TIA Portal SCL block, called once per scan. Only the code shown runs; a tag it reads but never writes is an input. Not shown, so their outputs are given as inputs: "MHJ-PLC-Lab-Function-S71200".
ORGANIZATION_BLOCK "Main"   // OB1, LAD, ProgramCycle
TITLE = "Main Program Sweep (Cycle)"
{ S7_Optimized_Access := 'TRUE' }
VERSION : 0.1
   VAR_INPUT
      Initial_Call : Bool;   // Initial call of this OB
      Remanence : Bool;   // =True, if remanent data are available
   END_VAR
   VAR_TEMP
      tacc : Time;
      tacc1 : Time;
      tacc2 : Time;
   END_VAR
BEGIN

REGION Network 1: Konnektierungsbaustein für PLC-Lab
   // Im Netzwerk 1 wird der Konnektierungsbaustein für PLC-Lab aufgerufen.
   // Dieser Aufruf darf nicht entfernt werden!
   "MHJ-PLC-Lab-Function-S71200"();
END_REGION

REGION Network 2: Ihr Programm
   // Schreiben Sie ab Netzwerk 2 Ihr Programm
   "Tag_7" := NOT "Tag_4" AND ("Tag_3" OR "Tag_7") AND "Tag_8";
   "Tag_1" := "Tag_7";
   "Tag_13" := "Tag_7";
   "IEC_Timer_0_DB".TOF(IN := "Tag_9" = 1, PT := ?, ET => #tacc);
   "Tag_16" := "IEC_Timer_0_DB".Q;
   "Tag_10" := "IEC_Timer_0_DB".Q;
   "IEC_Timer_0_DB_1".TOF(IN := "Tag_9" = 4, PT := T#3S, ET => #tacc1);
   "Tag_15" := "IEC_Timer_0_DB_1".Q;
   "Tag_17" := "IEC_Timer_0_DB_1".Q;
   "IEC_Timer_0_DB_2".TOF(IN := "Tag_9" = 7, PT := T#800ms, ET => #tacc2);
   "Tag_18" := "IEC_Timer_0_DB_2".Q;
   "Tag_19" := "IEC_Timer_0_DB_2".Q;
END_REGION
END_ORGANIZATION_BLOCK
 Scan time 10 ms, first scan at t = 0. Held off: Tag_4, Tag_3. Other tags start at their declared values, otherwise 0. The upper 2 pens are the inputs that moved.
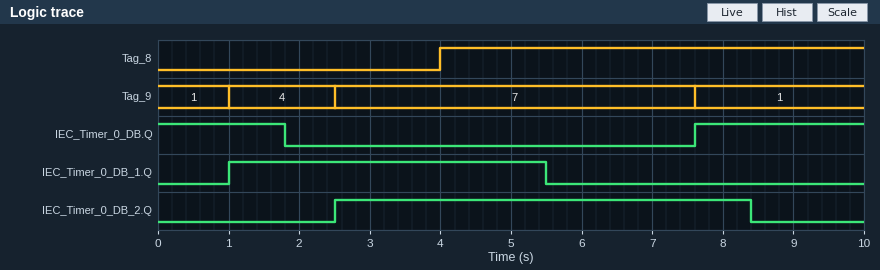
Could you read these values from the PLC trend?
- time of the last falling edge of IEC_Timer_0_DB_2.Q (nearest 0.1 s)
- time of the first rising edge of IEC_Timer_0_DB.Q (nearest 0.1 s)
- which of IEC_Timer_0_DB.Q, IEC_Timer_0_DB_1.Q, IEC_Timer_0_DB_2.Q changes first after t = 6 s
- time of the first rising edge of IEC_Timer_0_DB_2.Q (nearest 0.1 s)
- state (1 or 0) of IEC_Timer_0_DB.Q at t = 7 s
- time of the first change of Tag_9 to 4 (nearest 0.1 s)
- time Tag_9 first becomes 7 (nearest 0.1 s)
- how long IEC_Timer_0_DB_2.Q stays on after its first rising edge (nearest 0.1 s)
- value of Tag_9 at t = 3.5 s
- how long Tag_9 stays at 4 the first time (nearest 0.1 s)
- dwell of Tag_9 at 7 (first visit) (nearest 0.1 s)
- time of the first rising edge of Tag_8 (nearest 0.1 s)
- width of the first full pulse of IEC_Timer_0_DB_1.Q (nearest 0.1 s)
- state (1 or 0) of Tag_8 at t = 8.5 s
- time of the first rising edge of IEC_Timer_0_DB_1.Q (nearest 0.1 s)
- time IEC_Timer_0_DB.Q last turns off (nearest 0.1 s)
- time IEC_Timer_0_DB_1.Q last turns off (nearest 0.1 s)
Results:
8.4 s
7.6 s
IEC_Timer_0_DB.Q
2.5 s
0
1.0 s
2.5 s
5.9 s
7
1.5 s
5.1 s
4.0 s
4.5 s
1
1.0 s
1.8 s
5.5 s
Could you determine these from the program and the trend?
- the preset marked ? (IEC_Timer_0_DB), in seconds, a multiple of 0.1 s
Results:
0.8 s
